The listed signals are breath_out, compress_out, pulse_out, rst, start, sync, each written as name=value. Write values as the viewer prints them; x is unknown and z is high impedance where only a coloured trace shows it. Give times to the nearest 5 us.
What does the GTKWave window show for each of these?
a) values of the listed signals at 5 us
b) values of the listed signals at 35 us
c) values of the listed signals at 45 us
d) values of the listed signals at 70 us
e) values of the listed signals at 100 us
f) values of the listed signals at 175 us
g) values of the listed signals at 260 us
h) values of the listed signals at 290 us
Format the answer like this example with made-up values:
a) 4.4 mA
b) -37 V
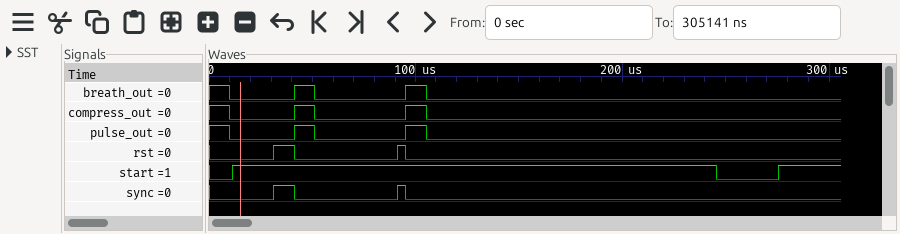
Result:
a) breath_out=1, compress_out=1, pulse_out=1, rst=0, start=0, sync=0
b) breath_out=0, compress_out=0, pulse_out=0, rst=1, start=1, sync=1
c) breath_out=1, compress_out=1, pulse_out=1, rst=0, start=1, sync=0
d) breath_out=0, compress_out=0, pulse_out=0, rst=0, start=1, sync=0
e) breath_out=1, compress_out=1, pulse_out=1, rst=0, start=1, sync=0
f) breath_out=0, compress_out=0, pulse_out=0, rst=0, start=1, sync=0
g) breath_out=0, compress_out=0, pulse_out=0, rst=0, start=0, sync=0
h) breath_out=0, compress_out=0, pulse_out=0, rst=0, start=1, sync=0
